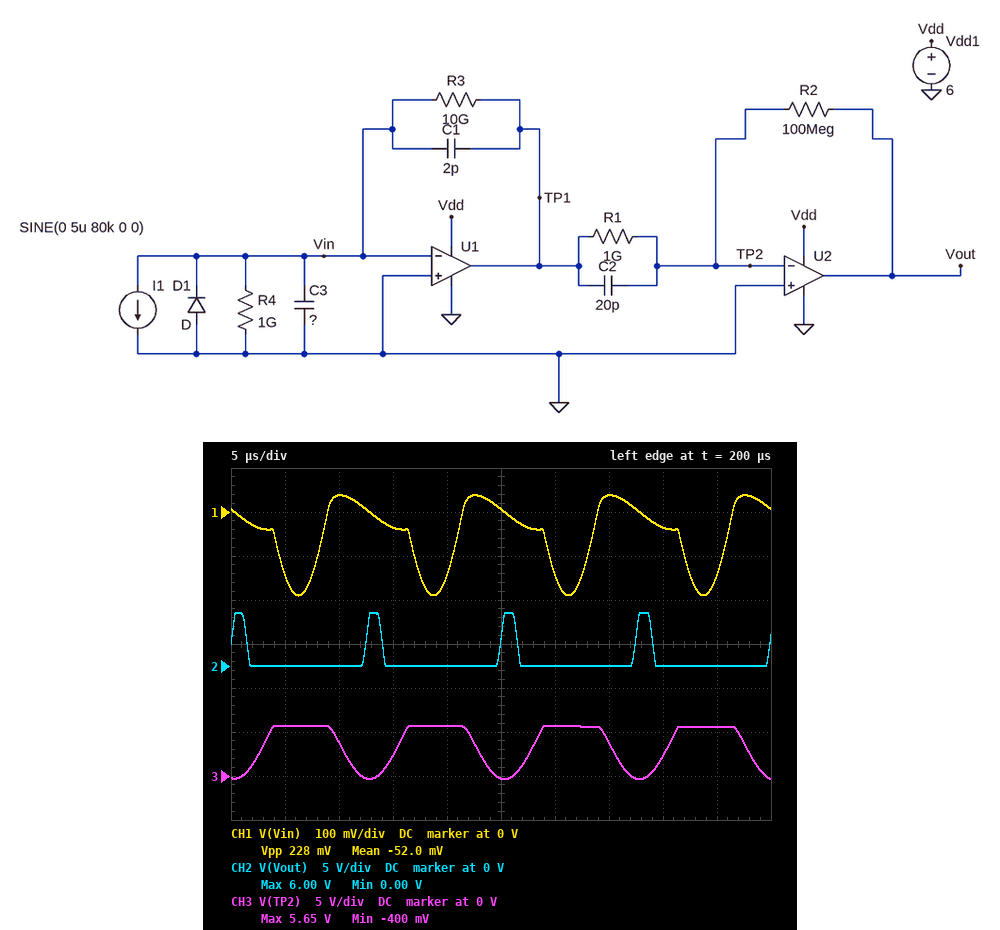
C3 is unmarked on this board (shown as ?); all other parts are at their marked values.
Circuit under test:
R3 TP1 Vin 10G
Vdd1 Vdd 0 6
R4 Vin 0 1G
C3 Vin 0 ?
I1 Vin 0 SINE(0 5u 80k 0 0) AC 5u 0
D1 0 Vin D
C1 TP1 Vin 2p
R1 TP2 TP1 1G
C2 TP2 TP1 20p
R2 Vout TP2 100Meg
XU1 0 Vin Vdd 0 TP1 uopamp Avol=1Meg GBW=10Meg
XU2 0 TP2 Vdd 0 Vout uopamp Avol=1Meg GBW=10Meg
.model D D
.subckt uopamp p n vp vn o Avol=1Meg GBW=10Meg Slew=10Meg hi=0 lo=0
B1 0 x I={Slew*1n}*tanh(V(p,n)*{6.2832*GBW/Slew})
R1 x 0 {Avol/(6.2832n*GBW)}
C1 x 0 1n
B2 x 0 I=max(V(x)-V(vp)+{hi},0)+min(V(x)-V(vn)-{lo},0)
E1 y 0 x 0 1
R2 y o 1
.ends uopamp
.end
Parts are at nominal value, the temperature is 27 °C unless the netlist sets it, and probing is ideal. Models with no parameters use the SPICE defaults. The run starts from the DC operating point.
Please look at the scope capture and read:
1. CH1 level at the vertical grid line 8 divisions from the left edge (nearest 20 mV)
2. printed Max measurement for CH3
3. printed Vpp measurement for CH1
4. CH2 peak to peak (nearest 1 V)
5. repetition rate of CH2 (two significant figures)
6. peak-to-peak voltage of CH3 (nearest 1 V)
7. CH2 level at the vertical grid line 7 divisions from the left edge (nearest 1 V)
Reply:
-40 mV
5.65 V
228 mV
6 V
80 kHz
6 V
0 V
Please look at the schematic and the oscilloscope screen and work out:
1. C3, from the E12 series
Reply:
39 pF
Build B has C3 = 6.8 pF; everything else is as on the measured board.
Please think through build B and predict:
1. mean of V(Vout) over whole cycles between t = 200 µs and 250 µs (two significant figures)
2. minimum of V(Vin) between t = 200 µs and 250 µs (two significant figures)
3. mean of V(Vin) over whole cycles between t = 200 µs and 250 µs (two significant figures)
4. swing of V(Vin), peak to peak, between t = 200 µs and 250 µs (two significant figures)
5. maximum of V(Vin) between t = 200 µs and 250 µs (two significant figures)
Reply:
1.9 V
-370 mV
46 mV
900 mV
530 mV
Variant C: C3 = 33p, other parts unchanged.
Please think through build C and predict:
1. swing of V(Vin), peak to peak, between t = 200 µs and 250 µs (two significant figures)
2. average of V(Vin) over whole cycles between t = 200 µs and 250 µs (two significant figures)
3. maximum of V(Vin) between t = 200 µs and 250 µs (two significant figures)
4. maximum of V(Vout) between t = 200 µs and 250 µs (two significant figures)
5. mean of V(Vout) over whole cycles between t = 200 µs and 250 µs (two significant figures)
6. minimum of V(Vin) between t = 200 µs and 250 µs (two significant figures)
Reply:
260 mV
-61 mV
39 mV
6.0 V
720 mV
-220 mV
